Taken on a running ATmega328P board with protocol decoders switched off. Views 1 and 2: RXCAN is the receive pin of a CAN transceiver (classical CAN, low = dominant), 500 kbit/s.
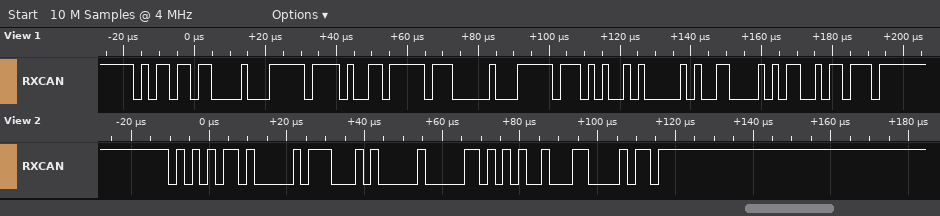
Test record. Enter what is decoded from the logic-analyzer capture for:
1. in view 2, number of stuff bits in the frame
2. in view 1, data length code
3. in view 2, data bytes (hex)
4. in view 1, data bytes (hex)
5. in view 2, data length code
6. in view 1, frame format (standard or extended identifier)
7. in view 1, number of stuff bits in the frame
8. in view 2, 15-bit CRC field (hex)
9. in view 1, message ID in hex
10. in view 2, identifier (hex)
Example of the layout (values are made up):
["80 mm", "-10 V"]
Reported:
["3", "8", "8A 00 55", "FF A6 FF 00 FF 52 81 30", "3", "standard", "5", "0x1185", "0x5B6", "0x55A"]
